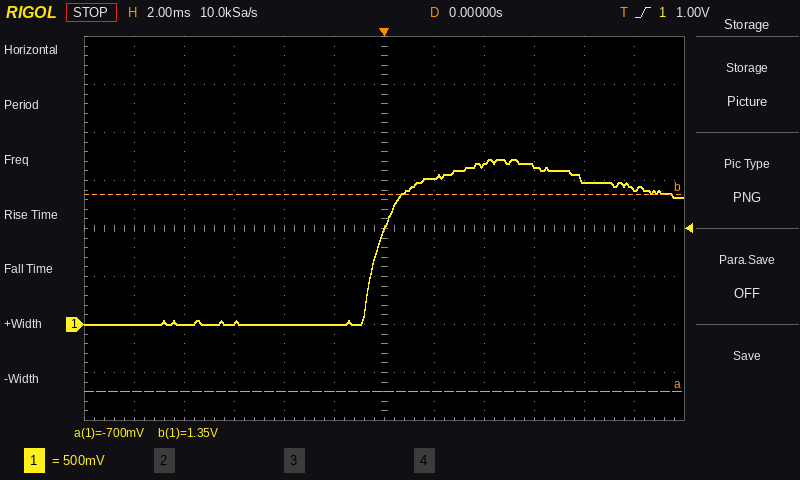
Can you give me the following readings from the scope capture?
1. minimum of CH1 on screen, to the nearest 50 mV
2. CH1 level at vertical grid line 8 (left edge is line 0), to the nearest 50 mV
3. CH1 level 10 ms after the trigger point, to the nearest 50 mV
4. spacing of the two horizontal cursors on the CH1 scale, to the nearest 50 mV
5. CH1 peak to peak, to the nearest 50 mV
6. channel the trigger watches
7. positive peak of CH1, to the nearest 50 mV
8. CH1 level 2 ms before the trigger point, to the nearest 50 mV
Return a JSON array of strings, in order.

["0 mV", "1.65 V", "1.40 V", "2.05 V", "1.70 V", "CH1", "1.70 V", "0 mV"]
